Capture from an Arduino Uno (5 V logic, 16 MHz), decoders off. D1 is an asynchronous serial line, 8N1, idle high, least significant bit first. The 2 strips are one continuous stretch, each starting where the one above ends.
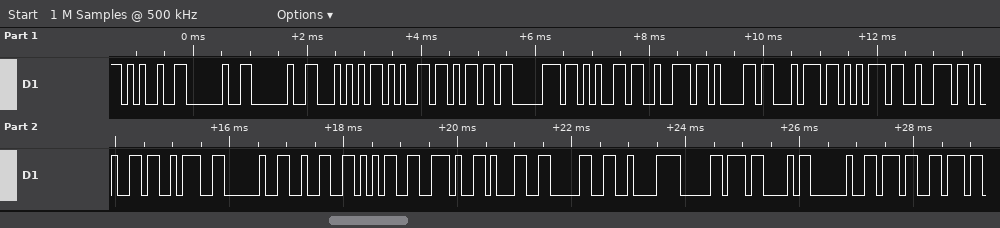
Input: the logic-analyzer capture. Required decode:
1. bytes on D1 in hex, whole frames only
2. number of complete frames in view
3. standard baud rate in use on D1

0x25 0x20 0x20 0x54 0x65 0x6D 0x70 0x65 0x72 0x61 0x74 0x75 0x72 0x65 0x3A 0x20 0x32 0x35 0x2E 0x31 0x30 0xC2 0xB0 0x43 0x20 0x37
26
9600 baud
